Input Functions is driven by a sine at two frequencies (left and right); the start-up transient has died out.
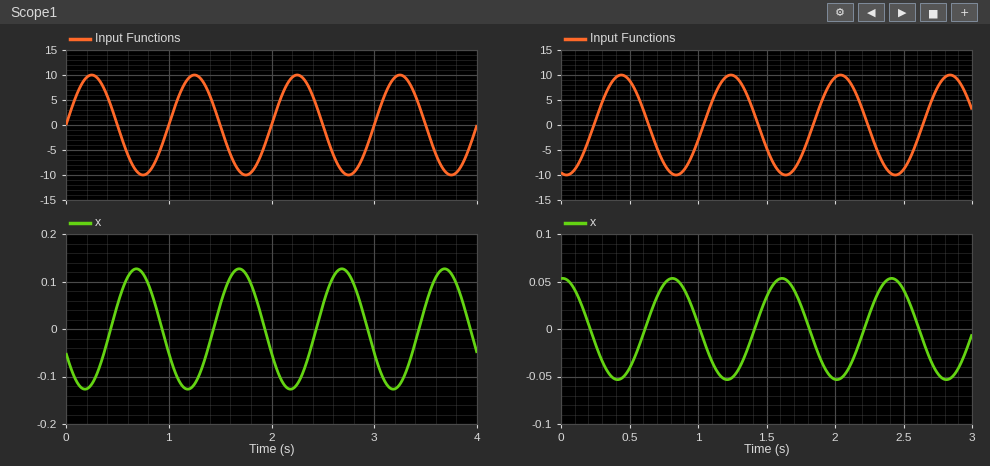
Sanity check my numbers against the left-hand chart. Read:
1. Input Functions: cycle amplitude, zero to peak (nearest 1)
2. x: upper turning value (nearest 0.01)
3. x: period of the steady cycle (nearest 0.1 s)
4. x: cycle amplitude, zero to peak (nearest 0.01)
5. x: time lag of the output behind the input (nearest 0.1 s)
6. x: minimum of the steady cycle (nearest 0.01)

10
0.13
1.0 s
0.13
0.4 s
-0.13
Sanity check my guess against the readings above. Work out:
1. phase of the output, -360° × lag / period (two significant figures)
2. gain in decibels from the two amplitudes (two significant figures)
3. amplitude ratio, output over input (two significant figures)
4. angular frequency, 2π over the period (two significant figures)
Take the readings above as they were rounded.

-140°
-38 dB
0.013
6.3 rad/s
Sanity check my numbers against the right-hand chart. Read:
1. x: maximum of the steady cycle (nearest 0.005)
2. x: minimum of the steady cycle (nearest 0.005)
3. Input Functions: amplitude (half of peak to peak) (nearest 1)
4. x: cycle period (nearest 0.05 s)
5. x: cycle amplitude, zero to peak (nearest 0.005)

0.055
-0.055
10
0.80 s
0.055
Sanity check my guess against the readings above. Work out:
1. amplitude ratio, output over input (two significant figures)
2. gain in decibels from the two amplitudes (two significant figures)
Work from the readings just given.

0.0055
-45 dB
